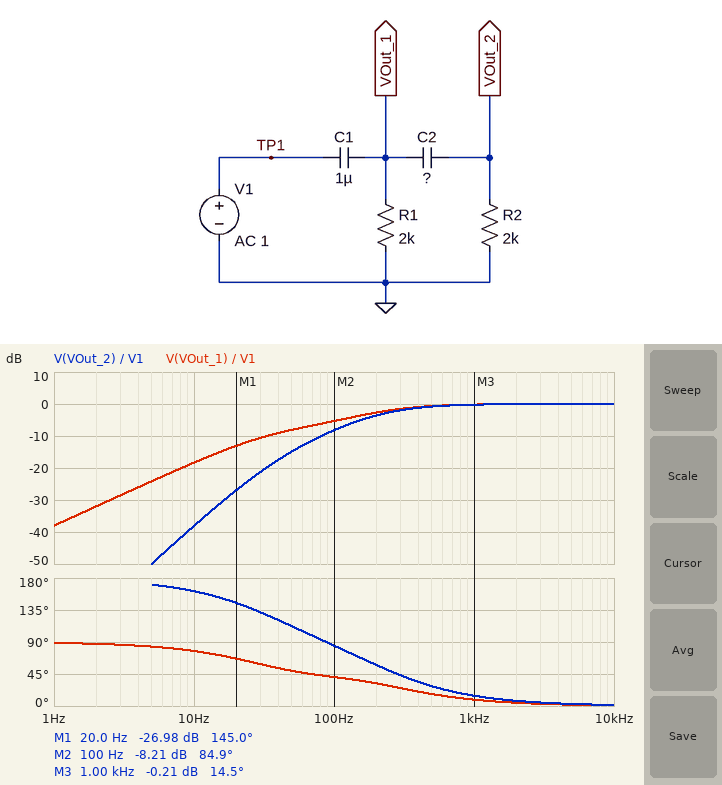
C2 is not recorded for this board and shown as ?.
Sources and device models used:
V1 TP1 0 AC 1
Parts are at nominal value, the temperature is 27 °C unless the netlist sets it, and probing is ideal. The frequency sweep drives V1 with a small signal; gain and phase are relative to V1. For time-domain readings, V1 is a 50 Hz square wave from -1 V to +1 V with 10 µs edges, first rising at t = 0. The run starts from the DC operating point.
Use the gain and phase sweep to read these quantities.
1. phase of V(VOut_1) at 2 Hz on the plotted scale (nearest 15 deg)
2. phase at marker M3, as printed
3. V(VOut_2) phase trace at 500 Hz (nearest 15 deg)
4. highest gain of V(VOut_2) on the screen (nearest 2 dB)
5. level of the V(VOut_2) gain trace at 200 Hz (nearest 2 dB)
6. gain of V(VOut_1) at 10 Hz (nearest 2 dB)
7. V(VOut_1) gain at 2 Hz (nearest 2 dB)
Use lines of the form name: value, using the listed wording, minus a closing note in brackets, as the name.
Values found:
phase of V(VOut_1) at 2 Hz on the plotted scale: 90 deg
phase at marker M3, as printed: 14.5 deg
V(VOut_2) phase trace at 500 Hz: 30 deg
highest gain of V(VOut_2) on the screen: 0 dB
level of the V(VOut_2) gain trace at 200 Hz: -4 dB
gain of V(VOut_1) at 10 Hz: -18 dB
V(VOut_1) gain at 2 Hz: -32 dB
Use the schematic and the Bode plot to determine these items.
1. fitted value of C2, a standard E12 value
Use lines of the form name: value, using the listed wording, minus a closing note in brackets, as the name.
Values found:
fitted value of C2, a standard E12 value: 820 nF
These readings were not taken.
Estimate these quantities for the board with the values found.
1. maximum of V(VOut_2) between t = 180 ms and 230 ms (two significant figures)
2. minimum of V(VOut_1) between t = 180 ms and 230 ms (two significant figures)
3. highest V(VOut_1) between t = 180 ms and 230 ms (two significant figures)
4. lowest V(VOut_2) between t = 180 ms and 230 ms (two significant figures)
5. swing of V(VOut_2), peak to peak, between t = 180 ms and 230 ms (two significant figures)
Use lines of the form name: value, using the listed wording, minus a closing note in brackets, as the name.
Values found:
maximum of V(VOut_2) between t = 180 ms and 230 ms: 2.0 V
minimum of V(VOut_1) between t = 180 ms and 230 ms: -1.9 V
highest V(VOut_1) between t = 180 ms and 230 ms: 1.9 V
lowest V(VOut_2) between t = 180 ms and 230 ms: -2.0 V
swing of V(VOut_2), peak to peak, between t = 180 ms and 230 ms: 4.0 V
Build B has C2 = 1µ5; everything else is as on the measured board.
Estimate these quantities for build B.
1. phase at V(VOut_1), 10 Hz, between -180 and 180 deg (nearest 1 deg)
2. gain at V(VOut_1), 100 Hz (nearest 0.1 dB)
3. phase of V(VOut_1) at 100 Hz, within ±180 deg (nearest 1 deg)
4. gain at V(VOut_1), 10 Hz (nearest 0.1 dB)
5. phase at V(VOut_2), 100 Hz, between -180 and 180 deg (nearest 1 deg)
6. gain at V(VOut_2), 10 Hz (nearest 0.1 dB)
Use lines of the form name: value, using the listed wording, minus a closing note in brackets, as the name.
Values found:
phase at V(VOut_1), 10 Hz, between -180 and 180 deg: 73 deg
gain at V(VOut_1), 100 Hz: -5.8 dB
phase of V(VOut_1) at 100 Hz, within ±180 deg: 47 deg
gain at V(VOut_1), 10 Hz: -18.7 dB
phase at V(VOut_2), 100 Hz, between -180 and 180 deg: 75 deg
gain at V(VOut_2), 10 Hz: -33.3 dB
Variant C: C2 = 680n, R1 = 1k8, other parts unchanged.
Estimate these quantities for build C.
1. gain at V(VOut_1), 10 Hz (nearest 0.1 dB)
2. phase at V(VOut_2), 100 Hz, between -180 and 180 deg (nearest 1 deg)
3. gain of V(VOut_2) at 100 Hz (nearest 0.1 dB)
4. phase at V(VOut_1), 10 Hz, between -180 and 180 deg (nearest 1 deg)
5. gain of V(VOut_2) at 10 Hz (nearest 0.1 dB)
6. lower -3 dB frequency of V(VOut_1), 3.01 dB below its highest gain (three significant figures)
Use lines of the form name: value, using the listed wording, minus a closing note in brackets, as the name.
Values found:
gain at V(VOut_1), 10 Hz: -19.1 dB
phase at V(VOut_2), 100 Hz, between -180 and 180 deg: 91 deg
gain of V(VOut_2) at 100 Hz: -9.1 dB
phase at V(VOut_1), 10 Hz, between -180 and 180 deg: 79 deg
gain of V(VOut_2) at 10 Hz: -40.5 dB
lower -3 dB frequency of V(VOut_1), 3.01 dB below its highest gain: 190 Hz
